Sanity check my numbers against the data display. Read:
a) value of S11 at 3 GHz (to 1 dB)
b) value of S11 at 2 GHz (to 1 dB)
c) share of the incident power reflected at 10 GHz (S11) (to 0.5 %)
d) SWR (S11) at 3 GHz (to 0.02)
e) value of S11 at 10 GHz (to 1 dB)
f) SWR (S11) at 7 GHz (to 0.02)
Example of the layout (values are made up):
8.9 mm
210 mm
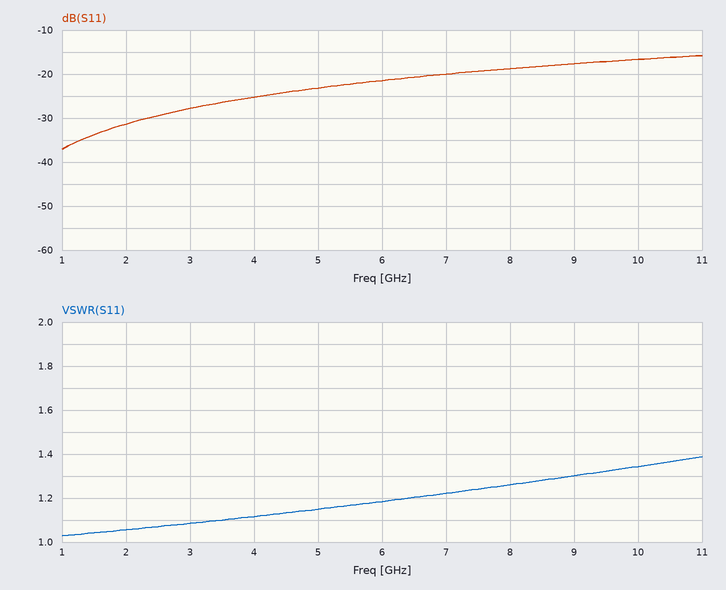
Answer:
-28 dB
-31 dB
2.0 %
1.08
-17 dB
1.22
